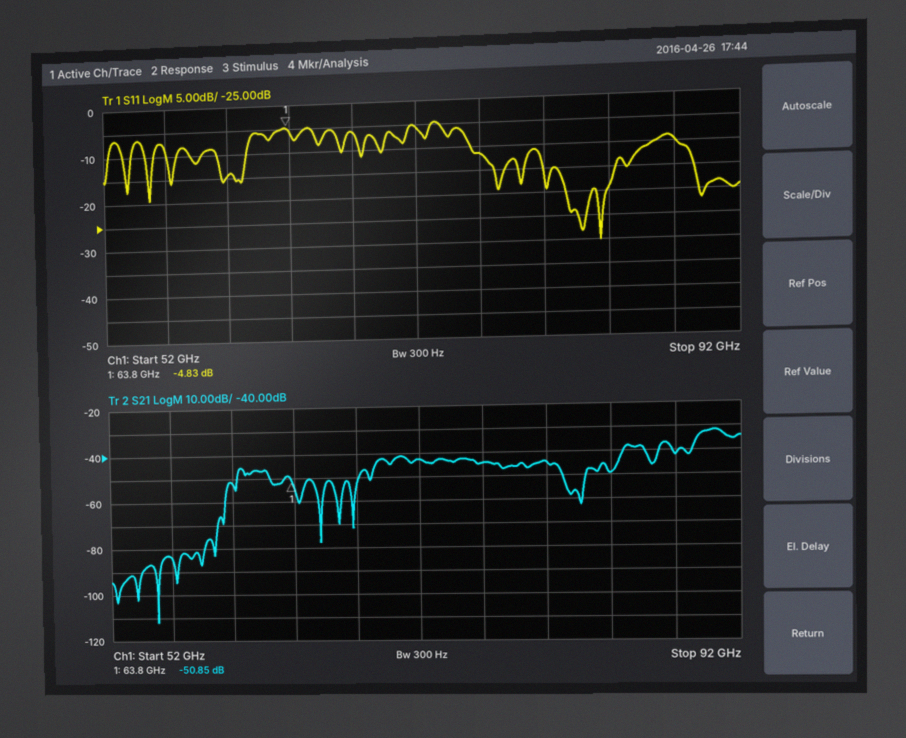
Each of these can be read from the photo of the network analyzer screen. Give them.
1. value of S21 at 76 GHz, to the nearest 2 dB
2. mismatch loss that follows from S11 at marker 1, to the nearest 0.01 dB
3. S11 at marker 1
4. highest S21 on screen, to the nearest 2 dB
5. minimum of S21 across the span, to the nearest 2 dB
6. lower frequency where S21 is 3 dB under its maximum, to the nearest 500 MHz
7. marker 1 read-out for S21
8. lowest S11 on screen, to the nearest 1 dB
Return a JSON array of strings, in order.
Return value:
["-44 dB", "1.73 dB", "-4.83 dB", "-32 dB", "-112 dB", "89.5 GHz", "-50.85 dB", "-30 dB"]
